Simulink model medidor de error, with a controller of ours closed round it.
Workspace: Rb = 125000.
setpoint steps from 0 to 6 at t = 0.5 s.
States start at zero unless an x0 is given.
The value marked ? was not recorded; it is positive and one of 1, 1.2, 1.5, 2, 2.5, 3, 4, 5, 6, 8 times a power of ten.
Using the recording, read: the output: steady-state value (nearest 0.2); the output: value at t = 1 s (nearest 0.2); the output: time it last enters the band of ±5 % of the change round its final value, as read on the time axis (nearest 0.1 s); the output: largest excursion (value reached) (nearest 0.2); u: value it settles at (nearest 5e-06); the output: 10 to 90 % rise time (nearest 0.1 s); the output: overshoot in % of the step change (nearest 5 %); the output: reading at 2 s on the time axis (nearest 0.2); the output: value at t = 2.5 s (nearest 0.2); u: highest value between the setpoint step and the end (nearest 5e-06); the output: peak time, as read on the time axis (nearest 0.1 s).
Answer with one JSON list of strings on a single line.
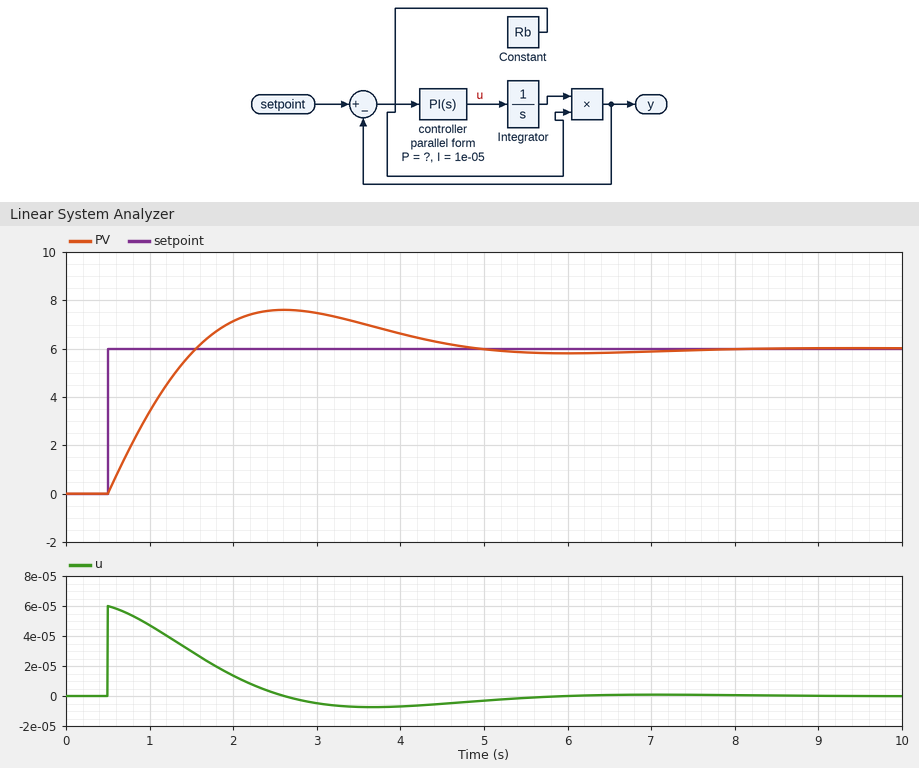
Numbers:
["6.0", "3.4", "4.4 s", "7.6", "0.000000", "0.8 s", "25 %", "7.2", "7.6", "0.000060", "2.6 s"]
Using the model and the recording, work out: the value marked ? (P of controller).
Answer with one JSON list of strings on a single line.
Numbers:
["1e-05"]
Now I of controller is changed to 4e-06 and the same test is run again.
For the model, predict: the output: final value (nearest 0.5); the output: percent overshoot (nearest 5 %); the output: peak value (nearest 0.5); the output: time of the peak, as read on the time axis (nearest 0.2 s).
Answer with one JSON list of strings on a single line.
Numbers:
["6.0", "15 %", "7.0", "3.4 s"]
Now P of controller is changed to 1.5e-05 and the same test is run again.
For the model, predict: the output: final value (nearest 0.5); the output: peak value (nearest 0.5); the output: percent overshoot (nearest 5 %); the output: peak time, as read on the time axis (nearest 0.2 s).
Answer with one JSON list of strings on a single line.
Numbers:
["6.0", "7.0", "15 %", "2.4 s"]
